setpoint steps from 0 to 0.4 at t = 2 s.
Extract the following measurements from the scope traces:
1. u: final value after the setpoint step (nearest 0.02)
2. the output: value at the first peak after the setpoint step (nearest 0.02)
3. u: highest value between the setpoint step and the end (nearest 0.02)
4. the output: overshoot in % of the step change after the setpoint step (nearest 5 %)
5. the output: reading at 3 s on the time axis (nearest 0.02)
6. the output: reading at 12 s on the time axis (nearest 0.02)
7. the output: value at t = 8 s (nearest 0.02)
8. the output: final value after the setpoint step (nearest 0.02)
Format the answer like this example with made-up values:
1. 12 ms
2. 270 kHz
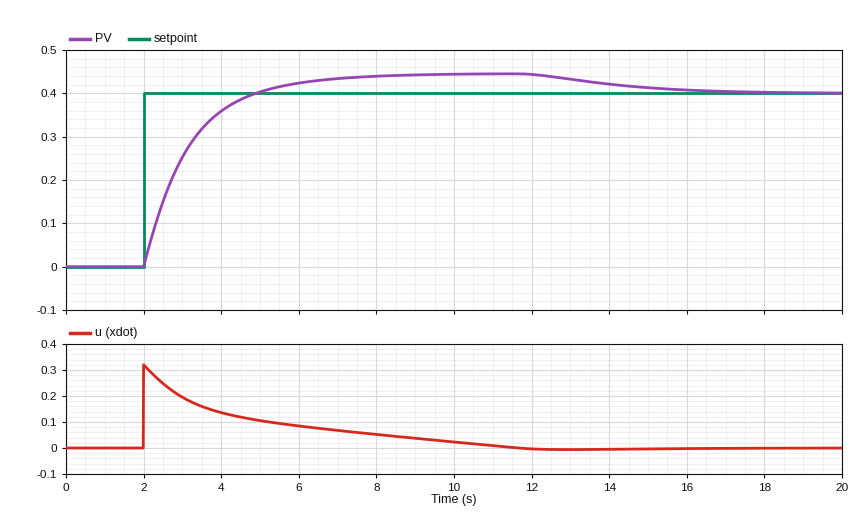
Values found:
1. 0.00
2. 0.44
3. 0.32
4. 10 %
5. 0.26
6. 0.44
7. 0.44
8. 0.40
